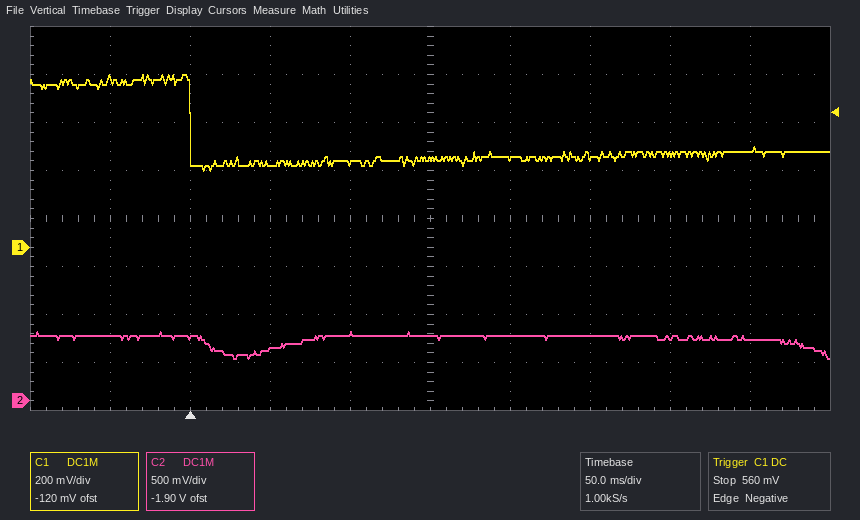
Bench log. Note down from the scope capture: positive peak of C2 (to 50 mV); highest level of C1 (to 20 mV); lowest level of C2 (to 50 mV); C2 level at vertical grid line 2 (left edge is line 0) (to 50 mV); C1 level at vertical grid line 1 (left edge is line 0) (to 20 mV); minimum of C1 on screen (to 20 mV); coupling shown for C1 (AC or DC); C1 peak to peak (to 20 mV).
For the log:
700 mV
720 mV
450 mV
650 mV
700 mV
320 mV
DC
400 mV
